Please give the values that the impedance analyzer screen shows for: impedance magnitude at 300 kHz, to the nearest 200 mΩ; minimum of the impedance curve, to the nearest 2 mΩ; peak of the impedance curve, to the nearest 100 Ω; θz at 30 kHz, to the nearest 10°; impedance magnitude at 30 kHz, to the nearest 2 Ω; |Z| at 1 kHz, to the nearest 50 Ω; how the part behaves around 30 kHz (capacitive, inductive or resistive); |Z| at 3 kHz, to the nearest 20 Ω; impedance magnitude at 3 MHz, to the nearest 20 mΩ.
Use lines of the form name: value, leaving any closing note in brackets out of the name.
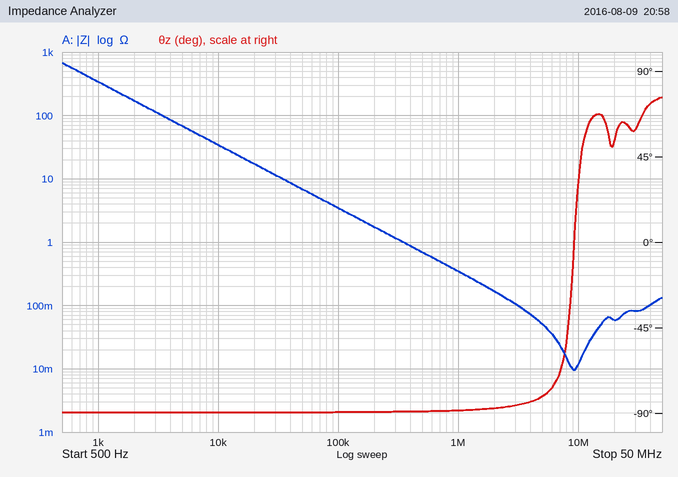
impedance magnitude at 300 kHz, to the nearest 200 mΩ: 1.2 Ω
minimum of the impedance curve, to the nearest 2 mΩ: 10 mΩ
peak of the impedance curve, to the nearest 100 Ω: 700 Ω
θz at 30 kHz, to the nearest 10°: -90°
impedance magnitude at 30 kHz, to the nearest 2 Ω: 12 Ω
|Z| at 1 kHz, to the nearest 50 Ω: 350 Ω
how the part behaves around 30 kHz: capacitive
|Z| at 3 kHz, to the nearest 20 Ω: 120 Ω
impedance magnitude at 3 MHz, to the nearest 20 mΩ: 100 mΩ
